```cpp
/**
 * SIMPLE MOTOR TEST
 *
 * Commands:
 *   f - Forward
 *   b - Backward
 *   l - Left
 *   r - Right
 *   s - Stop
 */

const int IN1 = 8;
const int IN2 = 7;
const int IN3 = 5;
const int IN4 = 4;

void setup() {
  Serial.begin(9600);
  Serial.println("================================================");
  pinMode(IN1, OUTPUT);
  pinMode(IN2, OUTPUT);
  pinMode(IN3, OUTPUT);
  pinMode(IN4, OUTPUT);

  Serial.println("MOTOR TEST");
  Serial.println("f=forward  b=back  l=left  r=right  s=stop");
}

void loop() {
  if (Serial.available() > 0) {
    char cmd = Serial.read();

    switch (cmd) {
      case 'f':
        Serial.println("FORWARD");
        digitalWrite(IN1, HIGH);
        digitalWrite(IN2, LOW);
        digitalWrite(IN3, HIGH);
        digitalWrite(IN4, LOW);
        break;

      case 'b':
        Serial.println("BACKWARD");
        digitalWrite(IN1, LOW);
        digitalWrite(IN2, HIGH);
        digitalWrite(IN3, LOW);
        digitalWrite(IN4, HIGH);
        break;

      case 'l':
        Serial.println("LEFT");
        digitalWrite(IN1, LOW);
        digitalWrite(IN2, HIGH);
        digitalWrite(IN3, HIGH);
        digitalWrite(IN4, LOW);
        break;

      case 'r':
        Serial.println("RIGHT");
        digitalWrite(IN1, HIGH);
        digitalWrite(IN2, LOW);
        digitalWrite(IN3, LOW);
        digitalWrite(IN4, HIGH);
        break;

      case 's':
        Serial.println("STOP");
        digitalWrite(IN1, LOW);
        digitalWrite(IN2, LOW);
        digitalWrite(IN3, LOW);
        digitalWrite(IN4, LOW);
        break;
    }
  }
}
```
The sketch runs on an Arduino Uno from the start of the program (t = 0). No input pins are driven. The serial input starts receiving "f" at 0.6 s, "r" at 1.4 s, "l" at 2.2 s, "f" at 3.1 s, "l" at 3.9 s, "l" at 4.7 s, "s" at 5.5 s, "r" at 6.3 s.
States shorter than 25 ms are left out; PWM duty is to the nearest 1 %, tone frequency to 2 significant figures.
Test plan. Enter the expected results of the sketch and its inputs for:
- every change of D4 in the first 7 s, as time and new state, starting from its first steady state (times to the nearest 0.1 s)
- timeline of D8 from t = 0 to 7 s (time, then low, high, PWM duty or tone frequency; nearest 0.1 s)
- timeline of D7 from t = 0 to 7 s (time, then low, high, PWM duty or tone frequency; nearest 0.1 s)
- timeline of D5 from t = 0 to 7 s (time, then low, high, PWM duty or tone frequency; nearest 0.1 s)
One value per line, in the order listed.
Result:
0 s low; 1.4 s high; 2.2 s low; 6.3 s high
0 s low; 0.6 s high; 2.2 s low; 3.1 s high; 3.9 s low; 6.3 s high
0 s low; 2.2 s high; 3.1 s low; 3.9 s high; 5.5 s low
0 s low; 0.6 s high; 1.4 s low; 2.2 s high; 5.5 s low
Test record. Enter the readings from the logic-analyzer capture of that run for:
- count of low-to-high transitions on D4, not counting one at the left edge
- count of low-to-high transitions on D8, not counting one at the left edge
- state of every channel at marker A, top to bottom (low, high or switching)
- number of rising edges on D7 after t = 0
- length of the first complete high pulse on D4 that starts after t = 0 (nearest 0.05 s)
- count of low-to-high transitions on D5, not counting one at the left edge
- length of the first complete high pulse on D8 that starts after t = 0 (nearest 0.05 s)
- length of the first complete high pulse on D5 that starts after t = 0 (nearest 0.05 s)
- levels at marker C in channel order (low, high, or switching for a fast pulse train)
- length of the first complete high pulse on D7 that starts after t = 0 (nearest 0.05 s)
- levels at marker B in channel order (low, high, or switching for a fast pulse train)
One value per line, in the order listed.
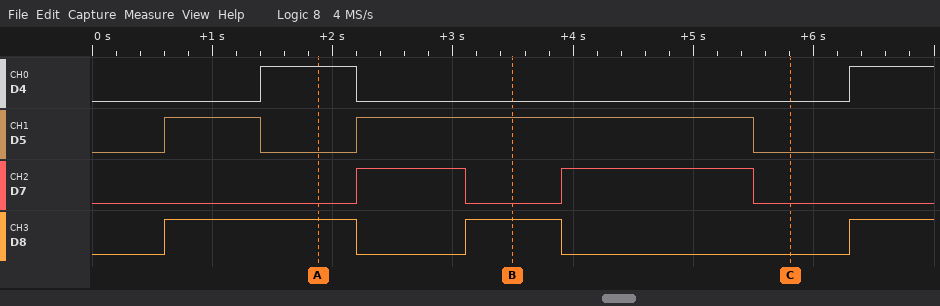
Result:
2
3
D4 high, D5 low, D7 low, D8 high
2
0.80 s
2
1.60 s
0.80 s
D4 low, D5 low, D7 low, D8 low
0.90 s
D4 low, D5 high, D7 low, D8 high
